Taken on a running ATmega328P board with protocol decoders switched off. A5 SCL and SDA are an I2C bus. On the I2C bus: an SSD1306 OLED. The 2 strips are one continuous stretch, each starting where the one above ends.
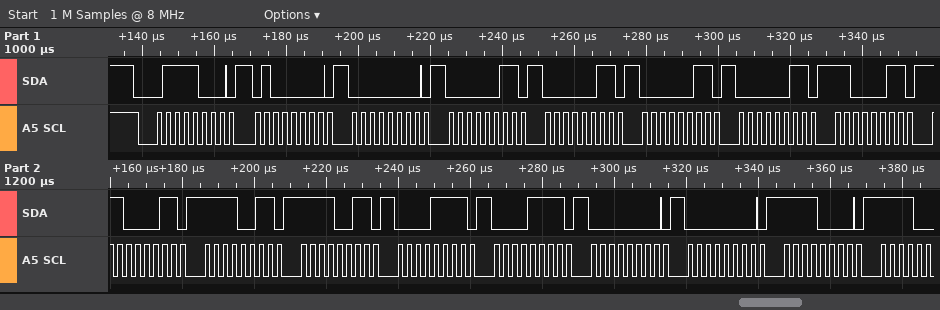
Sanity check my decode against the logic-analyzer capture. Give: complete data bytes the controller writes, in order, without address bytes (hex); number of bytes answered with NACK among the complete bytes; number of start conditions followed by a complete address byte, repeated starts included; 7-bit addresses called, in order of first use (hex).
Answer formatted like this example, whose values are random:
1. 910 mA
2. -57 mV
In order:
1. 40 00 03 03 03 03 C3 C3 F3 F3 0F 0F 00 00 F0
2. 0
3. 1
4. 0x3C
